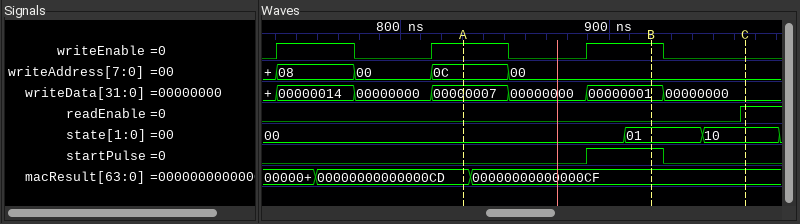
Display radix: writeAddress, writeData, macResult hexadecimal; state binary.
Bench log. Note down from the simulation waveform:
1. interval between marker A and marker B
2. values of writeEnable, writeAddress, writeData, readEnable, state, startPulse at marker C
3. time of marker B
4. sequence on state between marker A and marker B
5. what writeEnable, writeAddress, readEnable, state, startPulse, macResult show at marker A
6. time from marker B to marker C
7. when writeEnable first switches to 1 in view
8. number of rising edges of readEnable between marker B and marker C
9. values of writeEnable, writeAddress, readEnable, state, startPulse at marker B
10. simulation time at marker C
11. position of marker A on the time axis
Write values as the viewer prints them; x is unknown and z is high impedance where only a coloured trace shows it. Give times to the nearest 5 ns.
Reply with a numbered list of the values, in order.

1. 90 ns
2. writeEnable=0, writeAddress=00, writeData=00000000, readEnable=1, state=10, startPulse=0
3. 920 ns
4. 00, 01
5. writeEnable=1, writeAddress=0C, readEnable=0, state=00, startPulse=0, macResult=00000000000000CD
6. 45 ns
7. 740 ns
8. 1
9. writeEnable=1, writeAddress=00, readEnable=0, state=01, startPulse=1
10. 965 ns
11. 830 ns
